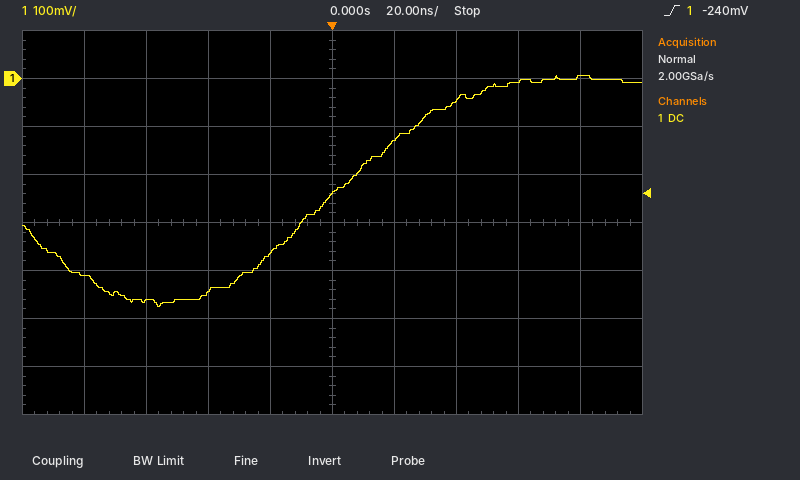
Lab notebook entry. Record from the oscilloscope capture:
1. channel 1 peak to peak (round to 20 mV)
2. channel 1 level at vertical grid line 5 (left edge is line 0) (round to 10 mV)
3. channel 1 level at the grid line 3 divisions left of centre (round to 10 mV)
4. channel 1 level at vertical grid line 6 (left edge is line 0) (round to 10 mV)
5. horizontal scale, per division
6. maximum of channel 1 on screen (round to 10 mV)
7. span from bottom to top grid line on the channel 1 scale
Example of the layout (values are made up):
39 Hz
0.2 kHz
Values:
480 mV
-240 mV
-460 mV
-130 mV
20 ns
10 mV
800 mV
